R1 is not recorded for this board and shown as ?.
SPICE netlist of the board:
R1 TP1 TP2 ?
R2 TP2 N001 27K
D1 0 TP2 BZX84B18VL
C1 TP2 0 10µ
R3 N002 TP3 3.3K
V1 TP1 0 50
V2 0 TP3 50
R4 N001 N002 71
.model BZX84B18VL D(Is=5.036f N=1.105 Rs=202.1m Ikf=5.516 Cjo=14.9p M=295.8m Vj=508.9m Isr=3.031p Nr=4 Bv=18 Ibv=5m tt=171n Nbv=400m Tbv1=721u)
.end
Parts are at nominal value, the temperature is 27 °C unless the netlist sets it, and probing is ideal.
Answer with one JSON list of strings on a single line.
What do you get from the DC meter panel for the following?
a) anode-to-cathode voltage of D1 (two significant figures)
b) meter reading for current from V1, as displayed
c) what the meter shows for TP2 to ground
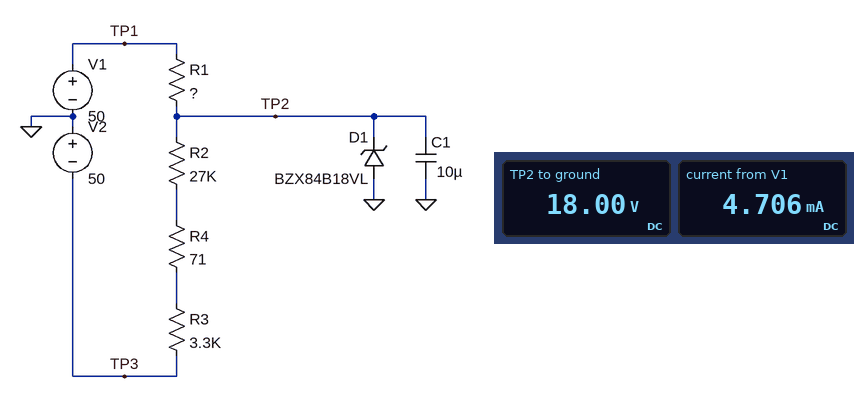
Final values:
["-18 V", "4.706 mA", "18.00 V"]
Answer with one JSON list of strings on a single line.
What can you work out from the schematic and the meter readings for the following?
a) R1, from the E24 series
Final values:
["6.8 kΩ"]
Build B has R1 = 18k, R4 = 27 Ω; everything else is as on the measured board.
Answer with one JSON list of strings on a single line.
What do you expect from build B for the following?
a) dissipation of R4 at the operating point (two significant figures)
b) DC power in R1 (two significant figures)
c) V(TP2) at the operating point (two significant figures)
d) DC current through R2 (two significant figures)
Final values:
["120 µW", "77 mW", "13 V", "2.1 mA"]
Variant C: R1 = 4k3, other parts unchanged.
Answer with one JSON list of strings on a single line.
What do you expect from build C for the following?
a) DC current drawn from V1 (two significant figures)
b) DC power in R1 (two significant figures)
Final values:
["7.4 mA", "240 mW"]
